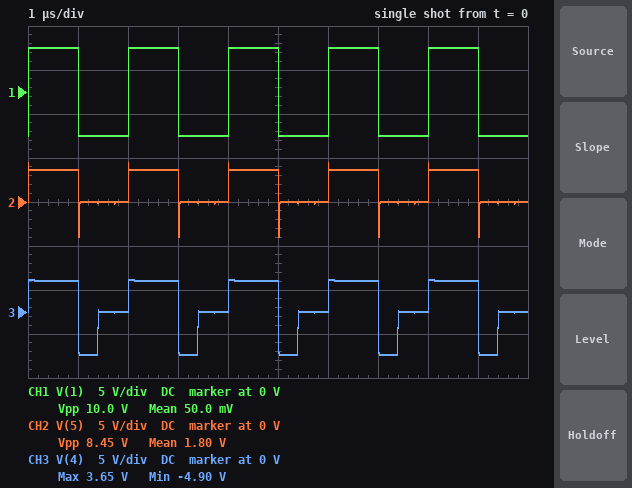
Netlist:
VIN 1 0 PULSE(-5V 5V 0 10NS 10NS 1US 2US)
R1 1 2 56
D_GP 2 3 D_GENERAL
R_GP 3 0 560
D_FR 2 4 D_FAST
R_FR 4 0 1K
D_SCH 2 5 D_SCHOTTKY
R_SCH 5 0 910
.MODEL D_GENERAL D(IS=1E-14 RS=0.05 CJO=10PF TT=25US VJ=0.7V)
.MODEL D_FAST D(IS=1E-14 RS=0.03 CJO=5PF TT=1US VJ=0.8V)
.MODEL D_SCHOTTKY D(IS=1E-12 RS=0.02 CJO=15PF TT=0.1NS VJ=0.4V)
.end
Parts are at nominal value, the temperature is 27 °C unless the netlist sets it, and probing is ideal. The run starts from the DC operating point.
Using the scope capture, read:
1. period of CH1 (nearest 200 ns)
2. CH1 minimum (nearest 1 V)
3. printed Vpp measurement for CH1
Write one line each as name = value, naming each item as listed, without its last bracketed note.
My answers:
period of CH1 = 2.0 µs
CH1 minimum = -5 V
printed Vpp measurement for CH1 = 10.0 V
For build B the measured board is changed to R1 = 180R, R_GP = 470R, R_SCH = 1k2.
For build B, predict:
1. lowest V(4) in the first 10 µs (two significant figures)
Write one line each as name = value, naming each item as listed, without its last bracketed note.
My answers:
lowest V(4) in the first 10 µs = -3.6 V
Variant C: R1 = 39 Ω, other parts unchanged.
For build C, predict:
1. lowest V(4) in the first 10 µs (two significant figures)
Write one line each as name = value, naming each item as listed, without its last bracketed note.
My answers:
lowest V(4) in the first 10 µs = -5.1 V
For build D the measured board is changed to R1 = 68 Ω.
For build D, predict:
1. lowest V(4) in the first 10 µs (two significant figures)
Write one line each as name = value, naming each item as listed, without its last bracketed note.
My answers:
lowest V(4) in the first 10 µs = -4.8 V
